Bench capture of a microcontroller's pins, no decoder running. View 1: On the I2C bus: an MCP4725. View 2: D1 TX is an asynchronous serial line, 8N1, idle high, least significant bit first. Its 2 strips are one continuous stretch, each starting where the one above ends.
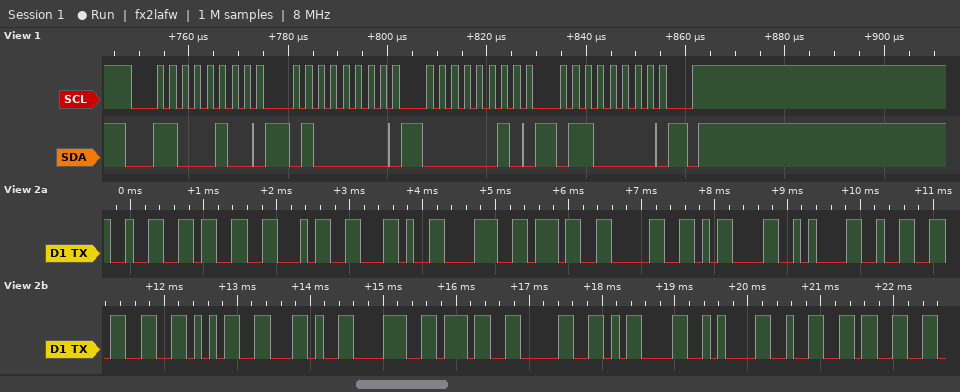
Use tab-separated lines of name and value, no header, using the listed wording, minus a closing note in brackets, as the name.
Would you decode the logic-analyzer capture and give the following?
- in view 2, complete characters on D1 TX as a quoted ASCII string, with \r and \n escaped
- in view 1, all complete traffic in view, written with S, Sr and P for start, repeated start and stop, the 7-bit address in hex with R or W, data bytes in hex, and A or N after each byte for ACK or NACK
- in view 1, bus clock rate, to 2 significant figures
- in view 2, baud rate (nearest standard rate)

in view 2, complete characters on D1 TX as a quoted ASCII string, with \r and \n escaped	"234,870\r\n235,870\r\n23"
in view 1, all complete traffic in view, written with S, Sr and P for start, repeated start and stop, the 7-bit address in hex with R or W, data bytes in hex, and A or N after each byte for ACK or NACK	S 62W A 40 A 02 A 60 A P
in view 1, bus clock rate, to 2 significant figures	400 kHz
in view 2, baud rate	9600 baud
